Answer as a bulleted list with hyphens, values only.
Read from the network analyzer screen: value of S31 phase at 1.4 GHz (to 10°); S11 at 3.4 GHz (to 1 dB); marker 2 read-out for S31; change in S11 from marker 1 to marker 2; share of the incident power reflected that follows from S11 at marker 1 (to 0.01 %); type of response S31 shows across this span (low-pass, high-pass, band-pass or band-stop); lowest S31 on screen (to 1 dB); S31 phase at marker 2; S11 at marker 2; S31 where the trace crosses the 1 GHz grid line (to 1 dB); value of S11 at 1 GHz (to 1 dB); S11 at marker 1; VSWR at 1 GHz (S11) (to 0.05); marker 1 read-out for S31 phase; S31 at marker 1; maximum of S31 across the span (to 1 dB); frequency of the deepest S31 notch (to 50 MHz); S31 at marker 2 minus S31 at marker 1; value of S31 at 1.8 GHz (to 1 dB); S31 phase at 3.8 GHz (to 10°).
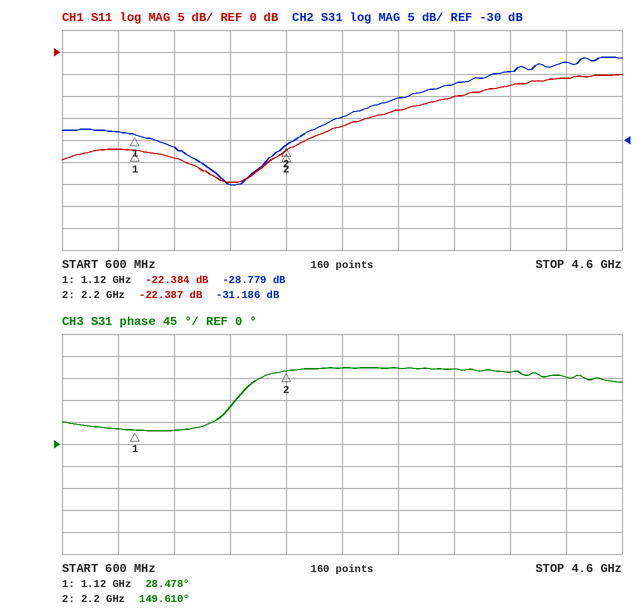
- 30°
- -10 dB
- -31.186 dB
- -0.003 dB
- 0.58 %
- high-pass
- -40 dB
- 149.610°
- -22.387 dB
- -28 dB
- -22 dB
- -22.384 dB
- 1.15
- 28.478°
- -28.779 dB
- -11 dB
- 1.85 GHz
- -2.407 dB
- -40 dB
- 150°
